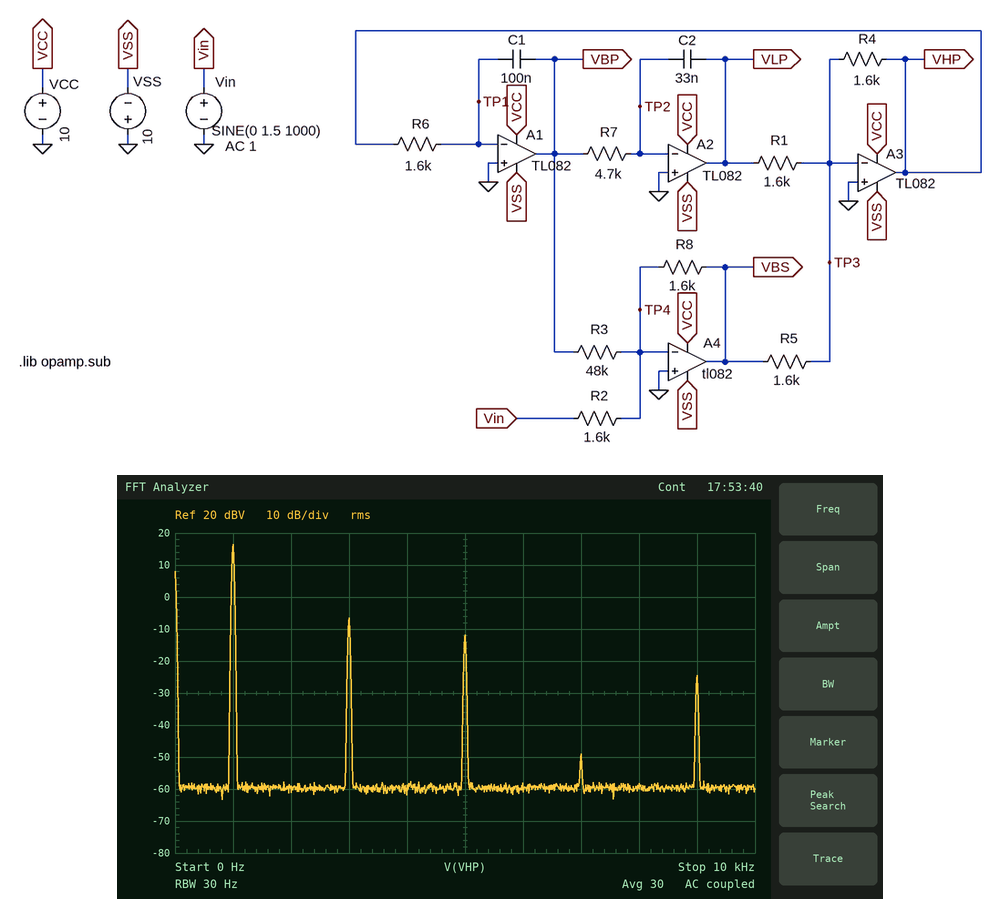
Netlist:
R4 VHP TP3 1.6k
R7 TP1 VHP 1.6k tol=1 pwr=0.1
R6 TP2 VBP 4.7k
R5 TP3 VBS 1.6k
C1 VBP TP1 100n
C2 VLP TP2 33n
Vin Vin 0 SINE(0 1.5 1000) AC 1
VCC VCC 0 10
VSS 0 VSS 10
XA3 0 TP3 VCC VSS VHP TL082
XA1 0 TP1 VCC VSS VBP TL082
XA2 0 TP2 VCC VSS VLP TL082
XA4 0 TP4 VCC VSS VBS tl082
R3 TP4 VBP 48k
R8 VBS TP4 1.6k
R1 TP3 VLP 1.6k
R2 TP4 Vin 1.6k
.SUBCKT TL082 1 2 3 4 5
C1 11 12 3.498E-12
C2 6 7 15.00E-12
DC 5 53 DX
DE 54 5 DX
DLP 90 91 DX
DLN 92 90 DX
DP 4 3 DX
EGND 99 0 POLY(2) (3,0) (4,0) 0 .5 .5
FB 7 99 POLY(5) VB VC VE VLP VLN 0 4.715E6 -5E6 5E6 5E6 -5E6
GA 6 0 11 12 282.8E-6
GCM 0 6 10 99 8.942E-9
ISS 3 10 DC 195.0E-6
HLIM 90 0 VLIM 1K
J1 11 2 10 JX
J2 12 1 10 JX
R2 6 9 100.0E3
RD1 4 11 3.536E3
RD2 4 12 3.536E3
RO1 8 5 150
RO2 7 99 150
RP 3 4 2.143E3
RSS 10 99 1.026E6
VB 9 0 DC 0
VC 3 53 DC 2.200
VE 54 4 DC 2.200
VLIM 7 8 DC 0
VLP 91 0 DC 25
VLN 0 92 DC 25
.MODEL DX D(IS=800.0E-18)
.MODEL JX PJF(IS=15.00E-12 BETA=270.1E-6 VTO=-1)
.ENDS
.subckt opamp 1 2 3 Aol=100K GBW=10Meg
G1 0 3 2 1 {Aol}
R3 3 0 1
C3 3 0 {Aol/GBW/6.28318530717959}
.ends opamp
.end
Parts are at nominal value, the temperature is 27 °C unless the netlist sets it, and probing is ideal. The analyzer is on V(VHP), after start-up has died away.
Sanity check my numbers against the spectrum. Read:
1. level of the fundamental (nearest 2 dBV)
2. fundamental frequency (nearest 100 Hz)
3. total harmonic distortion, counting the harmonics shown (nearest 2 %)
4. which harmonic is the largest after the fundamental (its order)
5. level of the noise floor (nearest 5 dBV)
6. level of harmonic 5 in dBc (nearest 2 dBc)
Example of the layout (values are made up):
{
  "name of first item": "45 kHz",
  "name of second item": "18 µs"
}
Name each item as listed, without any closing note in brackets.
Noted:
{
  "level of the fundamental": "16 dBV",
  "fundamental frequency": "1.0 kHz",
  "total harmonic distortion, counting the harmonics shown": "8 %",
  "which harmonic is the largest after the fundamental": "3",
  "level of the noise floor": "-60 dBV",
  "level of harmonic 5 in dBc": "-28 dBc"
}
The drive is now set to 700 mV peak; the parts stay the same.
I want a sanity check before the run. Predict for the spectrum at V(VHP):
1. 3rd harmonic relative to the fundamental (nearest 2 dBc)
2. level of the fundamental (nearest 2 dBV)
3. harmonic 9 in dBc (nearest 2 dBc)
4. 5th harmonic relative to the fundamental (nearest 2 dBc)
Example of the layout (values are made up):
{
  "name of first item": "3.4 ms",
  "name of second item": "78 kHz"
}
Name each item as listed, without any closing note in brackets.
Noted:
{
  "3rd harmonic relative to the fundamental": "-30 dBc",
  "level of the fundamental": "16 dBV",
  "harmonic 9 in dBc": "-50 dBc",
  "5th harmonic relative to the fundamental": "-32 dBc"
}
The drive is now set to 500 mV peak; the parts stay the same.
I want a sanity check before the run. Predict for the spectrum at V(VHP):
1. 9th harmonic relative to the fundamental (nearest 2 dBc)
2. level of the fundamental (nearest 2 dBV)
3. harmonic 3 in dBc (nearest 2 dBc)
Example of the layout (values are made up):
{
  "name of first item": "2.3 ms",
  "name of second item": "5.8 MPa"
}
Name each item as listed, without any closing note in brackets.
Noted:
{
  "9th harmonic relative to the fundamental": "-46 dBc",
  "level of the fundamental": "16 dBV",
  "harmonic 3 in dBc": "-34 dBc"
}
